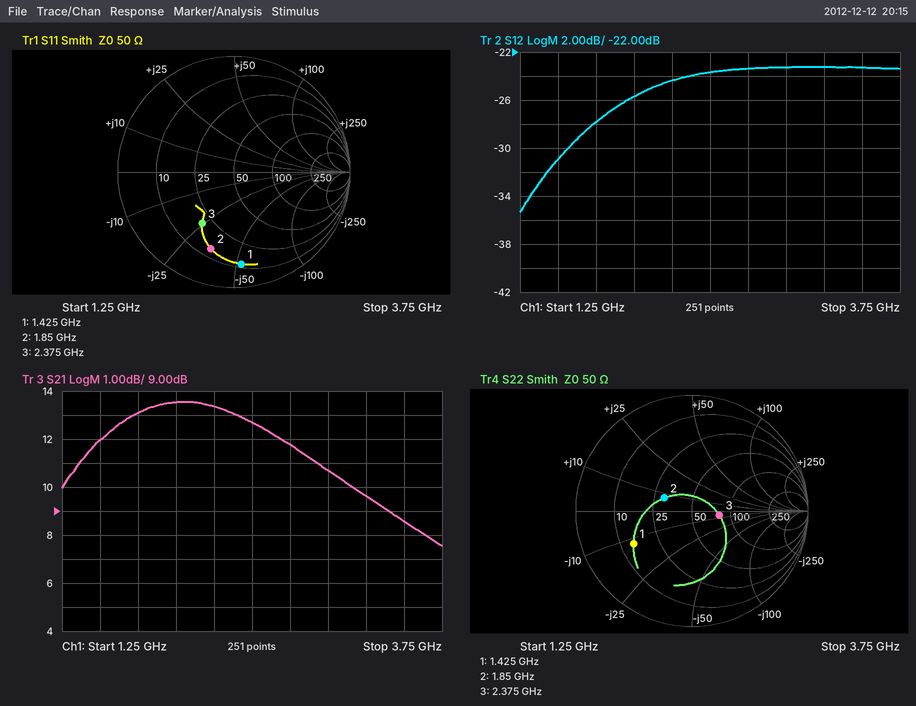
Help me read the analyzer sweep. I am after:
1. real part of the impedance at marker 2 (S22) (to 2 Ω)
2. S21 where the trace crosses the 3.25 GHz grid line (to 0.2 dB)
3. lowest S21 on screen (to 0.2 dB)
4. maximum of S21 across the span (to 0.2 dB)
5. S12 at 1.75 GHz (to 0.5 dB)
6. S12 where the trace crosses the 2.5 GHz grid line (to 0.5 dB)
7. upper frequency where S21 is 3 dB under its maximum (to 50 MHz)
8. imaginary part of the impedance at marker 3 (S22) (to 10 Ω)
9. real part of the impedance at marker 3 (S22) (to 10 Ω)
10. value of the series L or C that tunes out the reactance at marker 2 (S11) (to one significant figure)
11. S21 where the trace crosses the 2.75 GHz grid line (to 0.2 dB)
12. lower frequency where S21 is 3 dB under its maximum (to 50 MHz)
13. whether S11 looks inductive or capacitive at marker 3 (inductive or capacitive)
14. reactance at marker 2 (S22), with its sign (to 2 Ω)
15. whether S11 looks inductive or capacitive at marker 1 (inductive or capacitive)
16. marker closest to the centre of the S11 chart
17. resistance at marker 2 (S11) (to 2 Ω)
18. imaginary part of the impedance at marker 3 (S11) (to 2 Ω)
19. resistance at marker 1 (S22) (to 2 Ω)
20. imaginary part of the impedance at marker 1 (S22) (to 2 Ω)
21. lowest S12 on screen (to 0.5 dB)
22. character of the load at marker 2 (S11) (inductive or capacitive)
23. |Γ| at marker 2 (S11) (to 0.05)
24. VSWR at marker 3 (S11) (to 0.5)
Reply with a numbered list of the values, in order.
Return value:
1. 30 Ω
2. 9.6 dB
3. 7.6 dB
4. 13.6 dB
5. -28.0 dB
6. -23.5 dB
7. 3.05 GHz
8. -10 Ω
9. 80 Ω
10. 3 nH
11. 11.8 dB
12. 1.30 GHz
13. capacitive
14. +8 Ω
15. capacitive
16. marker 3
17. 14 Ω
18. -24 Ω
19. 14 Ω
20. -12 Ω
21. -35.5 dB
22. capacitive
23. 0.70
24. 3.0
